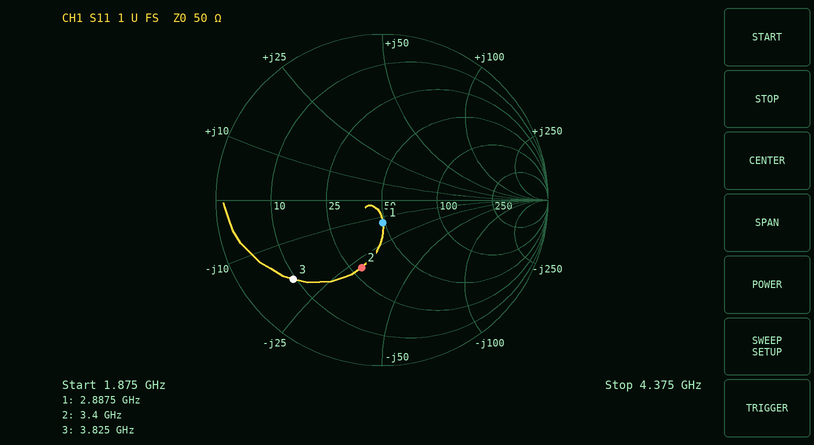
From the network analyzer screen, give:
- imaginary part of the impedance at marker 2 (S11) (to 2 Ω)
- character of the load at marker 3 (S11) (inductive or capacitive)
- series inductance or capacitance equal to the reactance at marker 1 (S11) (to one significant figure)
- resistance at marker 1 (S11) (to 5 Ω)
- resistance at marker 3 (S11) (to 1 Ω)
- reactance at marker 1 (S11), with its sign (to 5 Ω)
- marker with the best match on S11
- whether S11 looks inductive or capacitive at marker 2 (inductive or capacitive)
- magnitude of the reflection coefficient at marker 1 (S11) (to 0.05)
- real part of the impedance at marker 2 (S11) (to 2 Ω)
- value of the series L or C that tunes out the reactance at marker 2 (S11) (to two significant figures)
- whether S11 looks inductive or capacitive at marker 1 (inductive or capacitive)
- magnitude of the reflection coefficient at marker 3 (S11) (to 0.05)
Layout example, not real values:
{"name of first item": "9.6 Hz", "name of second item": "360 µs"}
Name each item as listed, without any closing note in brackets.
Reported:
{"imaginary part of the impedance at marker 2 (S11)": "-28 Ω", "character of the load at marker 3 (S11)": "capacitive", "series inductance or capacitance equal to the reactance at marker 1 (S11)": "4 pF", "resistance at marker 1 (S11)": "50 Ω", "resistance at marker 3 (S11)": "9 Ω", "reactance at marker 1 (S11), with its sign": "-15 Ω", "marker with the best match on S11": "marker 1", "whether S11 looks inductive or capacitive at marker 2": "capacitive", "magnitude of the reflection coefficient at marker 1 (S11)": "0.15", "real part of the impedance at marker 2 (S11)": "28 Ω", "value of the series L or C that tunes out the reactance at marker 2 (S11)": "1.3 nH", "whether S11 looks inductive or capacitive at marker 1": "capacitive", "magnitude of the reflection coefficient at marker 3 (S11)": "0.70"}
